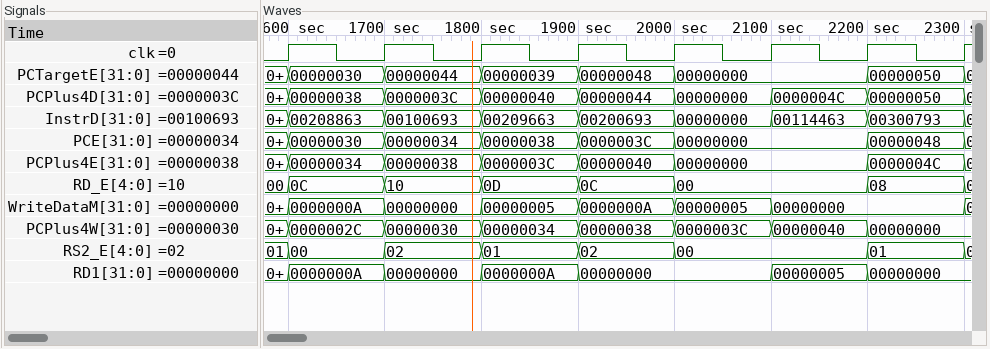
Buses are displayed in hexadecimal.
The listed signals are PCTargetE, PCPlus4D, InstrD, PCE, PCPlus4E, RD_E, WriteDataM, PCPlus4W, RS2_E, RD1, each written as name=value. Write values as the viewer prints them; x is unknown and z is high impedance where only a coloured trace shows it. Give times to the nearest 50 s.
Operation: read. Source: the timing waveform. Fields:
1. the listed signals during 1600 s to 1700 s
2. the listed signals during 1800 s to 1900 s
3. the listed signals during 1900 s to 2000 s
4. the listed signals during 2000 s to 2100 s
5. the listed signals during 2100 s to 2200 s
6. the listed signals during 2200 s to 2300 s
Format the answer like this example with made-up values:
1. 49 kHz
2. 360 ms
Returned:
1. PCTargetE=00000030, PCPlus4D=00000038, InstrD=00208863, PCE=00000030, PCPlus4E=00000034, RD_E=0C, WriteDataM=0000000A, PCPlus4W=0000002C, RS2_E=00, RD1=0000000A
2. PCTargetE=00000039, PCPlus4D=00000040, InstrD=00209663, PCE=00000038, PCPlus4E=0000003C, RD_E=0D, WriteDataM=00000005, PCPlus4W=00000034, RS2_E=01, RD1=0000000A
3. PCTargetE=00000048, PCPlus4D=00000044, InstrD=00200693, PCE=0000003C, PCPlus4E=00000040, RD_E=0C, WriteDataM=0000000A, PCPlus4W=00000038, RS2_E=02, RD1=00000000
4. PCTargetE=00000000, PCPlus4D=00000000, InstrD=00000000, PCE=00000000, PCPlus4E=00000000, RD_E=00, WriteDataM=00000005, PCPlus4W=0000003C, RS2_E=00, RD1=00000000
5. PCTargetE=00000000, PCPlus4D=0000004C, InstrD=00114463, PCE=00000000, PCPlus4E=00000000, RD_E=00, WriteDataM=00000000, PCPlus4W=00000040, RS2_E=00, RD1=00000005
6. PCTargetE=00000050, PCPlus4D=00000050, InstrD=00300793, PCE=00000048, PCPlus4E=0000004C, RD_E=08, WriteDataM=00000000, PCPlus4W=00000000, RS2_E=01, RD1=00000000
